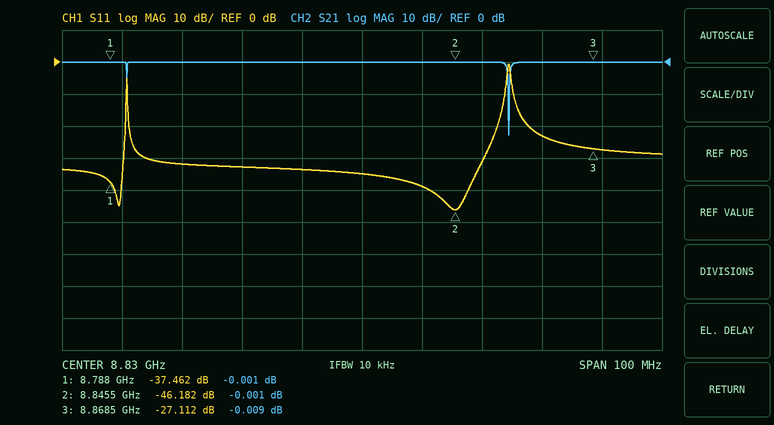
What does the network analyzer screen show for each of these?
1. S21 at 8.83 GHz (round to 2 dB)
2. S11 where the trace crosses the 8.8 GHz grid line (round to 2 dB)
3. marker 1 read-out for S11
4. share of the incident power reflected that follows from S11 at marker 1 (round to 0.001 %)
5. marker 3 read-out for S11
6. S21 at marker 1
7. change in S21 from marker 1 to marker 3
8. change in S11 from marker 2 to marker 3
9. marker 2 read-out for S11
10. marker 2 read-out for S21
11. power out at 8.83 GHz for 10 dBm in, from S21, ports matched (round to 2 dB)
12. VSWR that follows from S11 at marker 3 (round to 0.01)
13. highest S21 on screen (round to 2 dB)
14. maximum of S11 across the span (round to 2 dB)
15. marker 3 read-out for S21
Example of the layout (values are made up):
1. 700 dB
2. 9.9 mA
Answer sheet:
1. 0 dB
2. -32 dB
3. -37.462 dB
4. 0.018 %
5. -27.112 dB
6. -0.001 dB
7. -0.008 dB
8. 19.070 dB
9. -46.182 dB
10. -0.001 dB
11. 10 dBm
12. 1.09
13. 0 dB
14. 0 dB
15. -0.009 dB
